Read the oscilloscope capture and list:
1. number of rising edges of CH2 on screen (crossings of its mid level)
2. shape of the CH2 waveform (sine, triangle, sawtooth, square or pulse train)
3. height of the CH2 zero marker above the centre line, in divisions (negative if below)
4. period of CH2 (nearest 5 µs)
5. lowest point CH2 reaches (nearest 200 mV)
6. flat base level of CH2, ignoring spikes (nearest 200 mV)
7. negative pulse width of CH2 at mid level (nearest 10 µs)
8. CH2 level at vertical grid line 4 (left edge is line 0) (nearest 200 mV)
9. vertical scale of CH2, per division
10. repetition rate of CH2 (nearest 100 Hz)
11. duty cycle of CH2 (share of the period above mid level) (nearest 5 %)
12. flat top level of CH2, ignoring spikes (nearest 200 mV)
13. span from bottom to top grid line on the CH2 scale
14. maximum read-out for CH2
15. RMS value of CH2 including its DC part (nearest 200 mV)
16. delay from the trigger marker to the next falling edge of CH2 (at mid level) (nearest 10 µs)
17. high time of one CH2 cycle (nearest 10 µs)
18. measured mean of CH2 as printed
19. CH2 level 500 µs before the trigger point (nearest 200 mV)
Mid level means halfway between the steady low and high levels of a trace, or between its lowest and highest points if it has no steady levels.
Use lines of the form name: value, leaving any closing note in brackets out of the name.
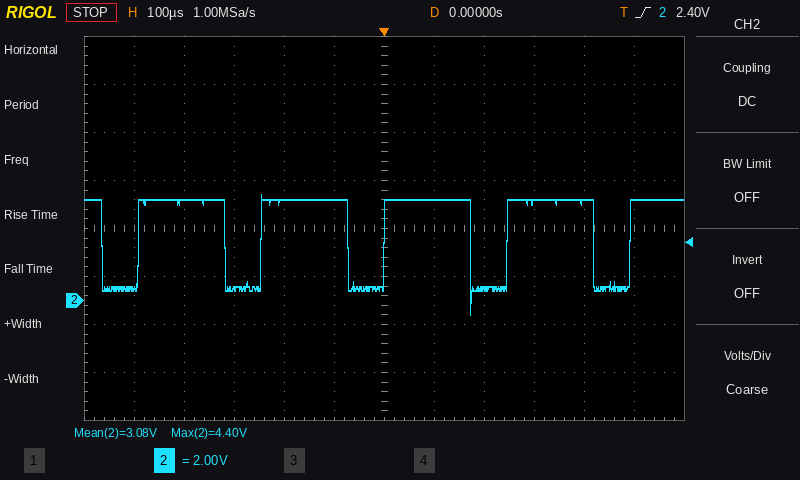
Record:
number of rising edges of CH2 on screen: 5
shape of the CH2 waveform: pulse train
height of the CH2 zero marker above the centre line, in divisions: -1.5 div
period of CH2: 245 µs
lowest point CH2 reaches: -600 mV
flat base level of CH2, ignoring spikes: 600 mV
negative pulse width of CH2 at mid level: 70 µs
CH2 level at vertical grid line 4 (left edge is line 0): 4.2 V
vertical scale of CH2, per division: 2 V
repetition rate of CH2: 4.1 kHz
duty cycle of CH2 (share of the period above mid level): 70 %
flat top level of CH2, ignoring spikes: 4.2 V
span from bottom to top grid line on the CH2 scale: 16 V
maximum read-out for CH2: 4.40 V
RMS value of CH2 including its DC part: 3.6 V
delay from the trigger marker to the next falling edge of CH2 (at mid level): 170 µs
high time of one CH2 cycle: 170 µs
measured mean of CH2 as printed: 3.08 V
CH2 level 500 µs before the trigger point: 600 mV
